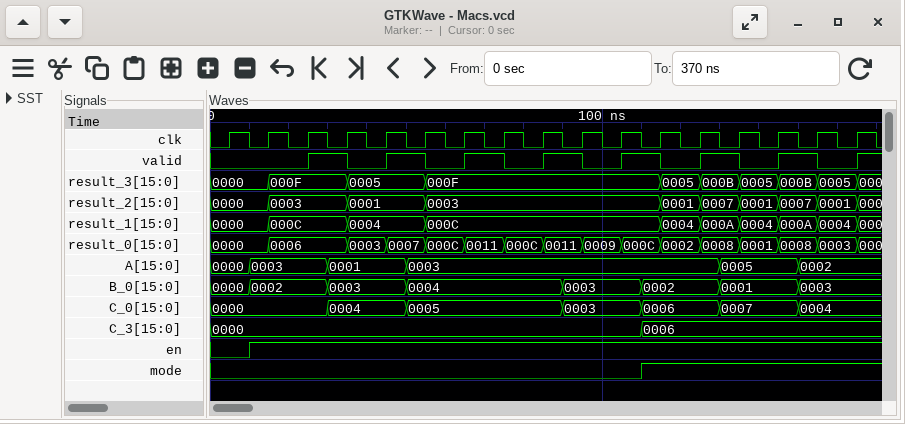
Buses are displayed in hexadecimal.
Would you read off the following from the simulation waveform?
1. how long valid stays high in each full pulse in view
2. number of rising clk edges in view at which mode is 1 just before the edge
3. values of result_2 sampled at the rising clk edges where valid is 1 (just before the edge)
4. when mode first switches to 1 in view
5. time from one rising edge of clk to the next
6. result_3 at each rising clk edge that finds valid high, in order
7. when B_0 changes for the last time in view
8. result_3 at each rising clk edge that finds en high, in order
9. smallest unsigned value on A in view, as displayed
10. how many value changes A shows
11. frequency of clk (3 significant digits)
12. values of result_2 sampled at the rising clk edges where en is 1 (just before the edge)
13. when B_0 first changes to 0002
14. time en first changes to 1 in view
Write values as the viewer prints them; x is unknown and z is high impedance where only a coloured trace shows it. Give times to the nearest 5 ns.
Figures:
10 ns, 10 ns, 10 ns, 10 ns, 10 ns, 10 ns, 10 ns
6
0003, 0001, 0003, 0003, 0003, 0007, 0007
110 ns
10 ns
000F, 0005, 000F, 000F, 000F, 000B, 000B
150 ns
0000, 000F, 000F, 0005, 0005, 000F, 000F, 000F, 000F, 000F, 000F, 0005, 000B, 0005, 000B, 0005
0000
5
100 MHz
0000, 0003, 0003, 0001, 0001, 0003, 0003, 0003, 0003, 0003, 0003, 0001, 0007, 0001, 0007, 0001
10 ns
10 ns
